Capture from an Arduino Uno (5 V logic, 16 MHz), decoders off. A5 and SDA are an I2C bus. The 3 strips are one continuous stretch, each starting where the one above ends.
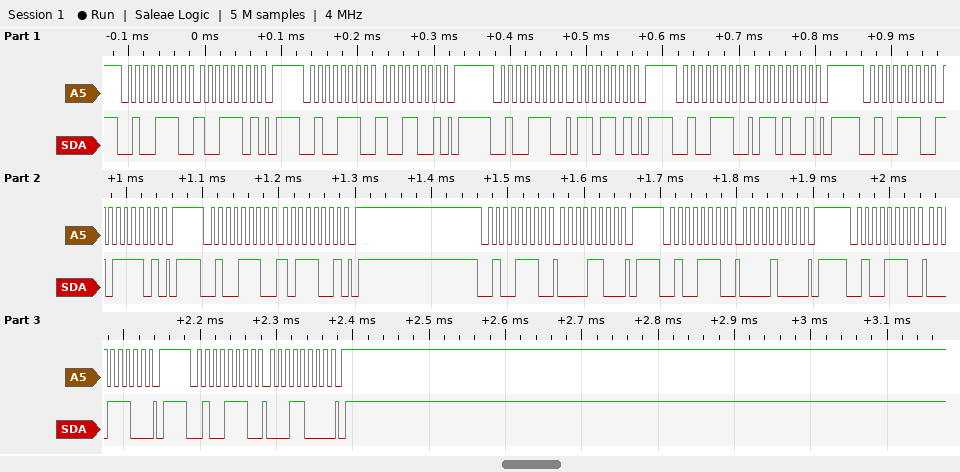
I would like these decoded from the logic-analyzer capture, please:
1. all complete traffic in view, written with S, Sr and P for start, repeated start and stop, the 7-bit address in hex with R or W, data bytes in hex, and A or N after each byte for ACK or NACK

S 27W A 9D A P S 27W A 99 A P S 27W A 6D A P S 27W A 69 A P S 27W A BD A P S 27W A B9 A P S 27W A 0C A P S 27W A 08 A P S 27W A 1C A P S 27W A 18 A P
